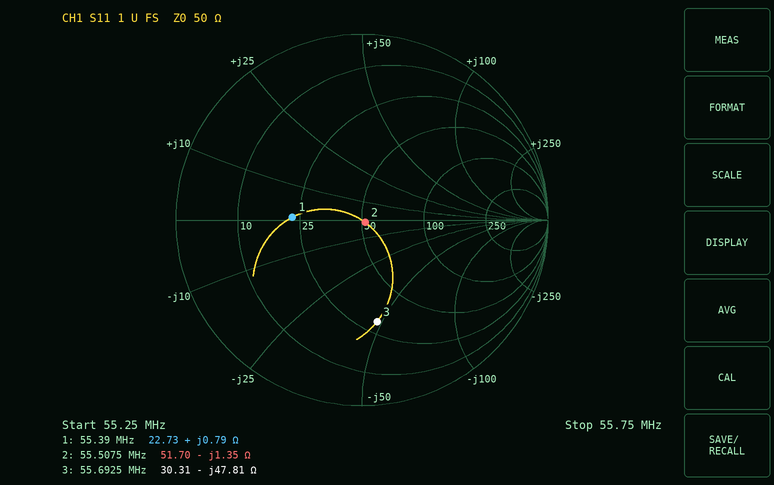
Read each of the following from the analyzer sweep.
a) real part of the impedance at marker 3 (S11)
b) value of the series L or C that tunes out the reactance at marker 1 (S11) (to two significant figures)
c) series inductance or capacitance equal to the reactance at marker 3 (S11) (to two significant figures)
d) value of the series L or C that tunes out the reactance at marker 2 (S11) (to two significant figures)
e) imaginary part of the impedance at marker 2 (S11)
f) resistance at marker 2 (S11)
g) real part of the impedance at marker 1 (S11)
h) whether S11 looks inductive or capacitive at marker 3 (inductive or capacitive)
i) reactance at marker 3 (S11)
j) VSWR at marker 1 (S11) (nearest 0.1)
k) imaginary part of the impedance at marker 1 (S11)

30.31 Ω
3.6 nF
60 pF
3.9 nH
-1.35 Ω
51.70 Ω
22.73 Ω
capacitive
-47.81 Ω
2.2
+0.79 Ω
